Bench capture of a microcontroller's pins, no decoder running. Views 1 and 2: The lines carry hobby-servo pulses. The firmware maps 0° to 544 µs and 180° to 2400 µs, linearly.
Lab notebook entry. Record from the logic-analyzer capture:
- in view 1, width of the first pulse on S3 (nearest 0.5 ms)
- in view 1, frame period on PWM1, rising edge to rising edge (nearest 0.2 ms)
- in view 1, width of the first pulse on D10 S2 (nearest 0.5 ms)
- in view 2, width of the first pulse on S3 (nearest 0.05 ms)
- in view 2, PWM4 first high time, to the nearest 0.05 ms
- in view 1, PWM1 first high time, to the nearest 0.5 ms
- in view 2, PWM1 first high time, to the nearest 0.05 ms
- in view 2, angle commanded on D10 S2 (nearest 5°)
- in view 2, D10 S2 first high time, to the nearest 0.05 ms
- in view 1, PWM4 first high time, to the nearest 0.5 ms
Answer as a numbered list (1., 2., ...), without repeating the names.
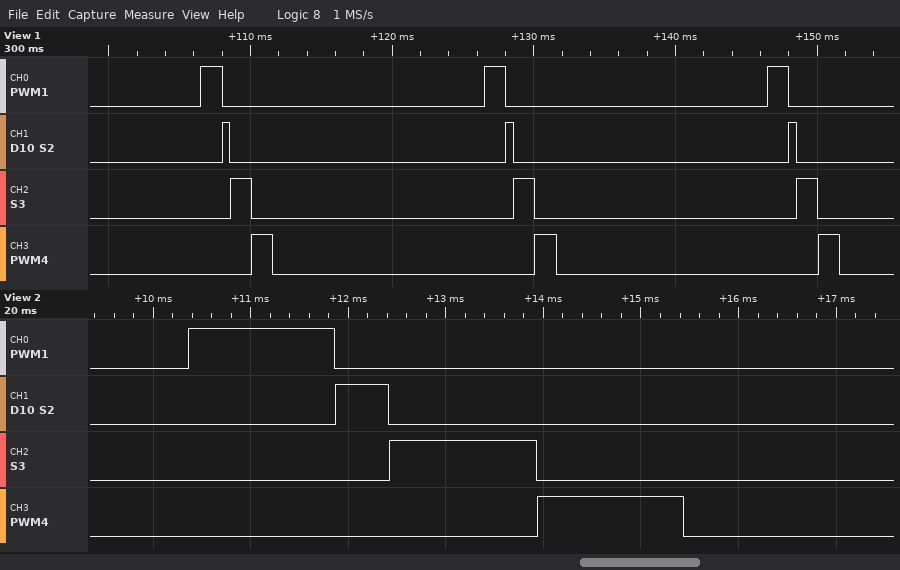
1. 1.5 ms
2. 20.0 ms
3. 0.5 ms
4. 1.50 ms
5. 1.50 ms
6. 1.5 ms
7. 1.50 ms
8. 0°
9. 0.55 ms
10. 1.5 ms
